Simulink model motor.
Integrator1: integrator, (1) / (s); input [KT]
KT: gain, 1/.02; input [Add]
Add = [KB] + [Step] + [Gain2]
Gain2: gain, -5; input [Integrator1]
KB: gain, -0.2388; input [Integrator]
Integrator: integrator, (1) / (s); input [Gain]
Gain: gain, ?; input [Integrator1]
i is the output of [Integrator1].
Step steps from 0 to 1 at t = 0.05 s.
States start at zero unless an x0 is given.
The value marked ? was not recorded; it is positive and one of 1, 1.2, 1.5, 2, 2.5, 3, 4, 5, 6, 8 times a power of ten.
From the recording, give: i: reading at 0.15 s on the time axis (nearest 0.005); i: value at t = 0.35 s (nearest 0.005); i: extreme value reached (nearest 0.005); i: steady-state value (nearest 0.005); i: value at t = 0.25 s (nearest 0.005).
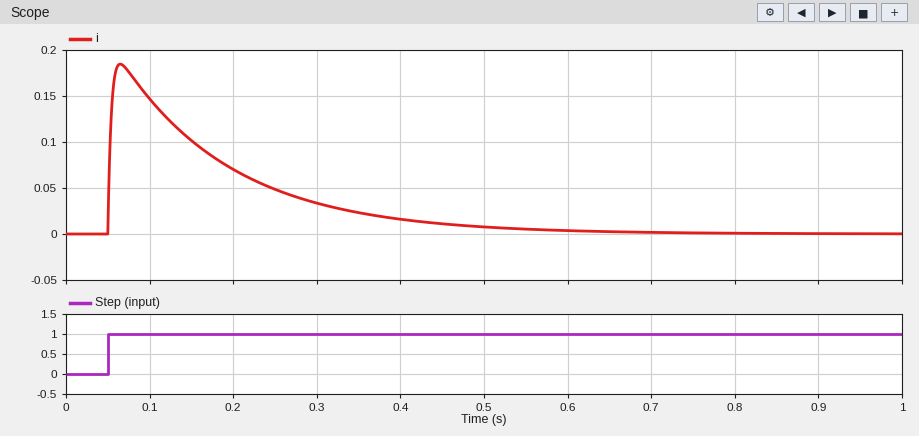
0.100
0.025
0.185
0.000
0.050
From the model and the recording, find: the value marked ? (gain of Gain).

150
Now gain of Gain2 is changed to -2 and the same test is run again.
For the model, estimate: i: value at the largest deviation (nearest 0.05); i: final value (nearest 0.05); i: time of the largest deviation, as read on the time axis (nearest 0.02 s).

0.40
0.00
0.08 s
